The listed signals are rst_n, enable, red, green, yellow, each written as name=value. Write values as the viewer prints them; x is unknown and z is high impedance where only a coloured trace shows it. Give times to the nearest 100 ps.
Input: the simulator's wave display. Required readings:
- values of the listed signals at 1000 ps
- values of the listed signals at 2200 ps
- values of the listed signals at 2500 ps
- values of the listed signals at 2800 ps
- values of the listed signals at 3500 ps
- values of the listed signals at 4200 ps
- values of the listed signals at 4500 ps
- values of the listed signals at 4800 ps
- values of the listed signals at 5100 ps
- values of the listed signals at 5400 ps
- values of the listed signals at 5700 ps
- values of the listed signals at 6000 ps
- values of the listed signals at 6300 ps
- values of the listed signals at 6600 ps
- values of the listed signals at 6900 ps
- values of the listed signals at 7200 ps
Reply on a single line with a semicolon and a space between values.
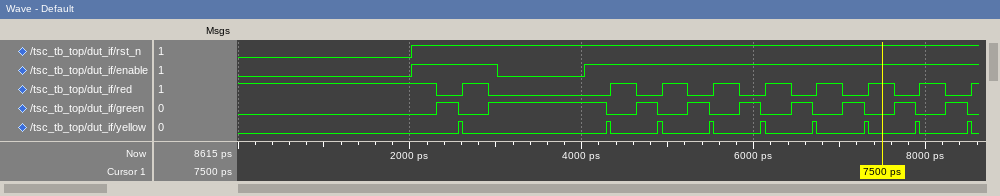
rst_n=0, enable=0, red=1, green=0, yellow=0; rst_n=1, enable=1, red=1, green=0, yellow=0; rst_n=1, enable=1, red=0, green=1, yellow=0; rst_n=1, enable=1, red=1, green=0, yellow=0; rst_n=1, enable=0, red=0, green=1, yellow=0; rst_n=1, enable=1, red=0, green=1, yellow=0; rst_n=1, enable=1, red=1, green=0, yellow=0; rst_n=1, enable=1, red=0, green=1, yellow=0; rst_n=1, enable=1, red=1, green=0, yellow=0; rst_n=1, enable=1, red=0, green=1, yellow=0; rst_n=1, enable=1, red=1, green=0, yellow=0; rst_n=1, enable=1, red=0, green=1, yellow=0; rst_n=1, enable=1, red=1, green=0, yellow=0; rst_n=1, enable=1, red=0, green=1, yellow=0; rst_n=1, enable=1, red=1, green=0, yellow=0; rst_n=1, enable=1, red=0, green=1, yellow=0
